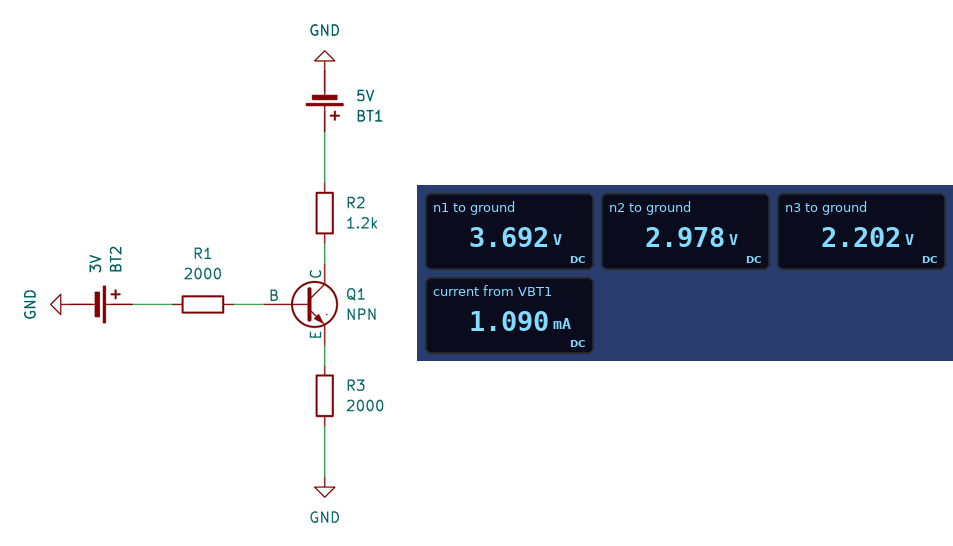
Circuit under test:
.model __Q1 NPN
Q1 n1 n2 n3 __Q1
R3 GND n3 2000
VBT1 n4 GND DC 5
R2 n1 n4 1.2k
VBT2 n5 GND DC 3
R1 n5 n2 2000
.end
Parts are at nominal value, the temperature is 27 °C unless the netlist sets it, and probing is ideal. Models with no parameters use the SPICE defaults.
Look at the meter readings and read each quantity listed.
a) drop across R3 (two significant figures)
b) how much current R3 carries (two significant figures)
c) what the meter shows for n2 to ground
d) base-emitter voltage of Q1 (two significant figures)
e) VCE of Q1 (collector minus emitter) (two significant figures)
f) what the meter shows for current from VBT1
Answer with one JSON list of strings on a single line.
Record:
["2.2 V", "1.1 mA", "2.978 V", "780 mV", "1.5 V", "1.090 mA"]
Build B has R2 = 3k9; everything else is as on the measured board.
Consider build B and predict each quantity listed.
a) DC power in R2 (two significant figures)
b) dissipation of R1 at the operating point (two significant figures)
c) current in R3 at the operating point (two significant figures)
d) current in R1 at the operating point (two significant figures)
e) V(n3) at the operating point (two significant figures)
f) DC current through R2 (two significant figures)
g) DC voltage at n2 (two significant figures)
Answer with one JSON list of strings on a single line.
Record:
["2.4 mW", "54 µW", "950 µA", "160 µA", "1.9 V", "780 µA", "2.7 V"]
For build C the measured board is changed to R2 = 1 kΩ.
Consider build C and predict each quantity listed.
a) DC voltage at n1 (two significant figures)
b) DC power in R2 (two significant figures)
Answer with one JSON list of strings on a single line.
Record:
["3.9 V", "1.2 mW"]
